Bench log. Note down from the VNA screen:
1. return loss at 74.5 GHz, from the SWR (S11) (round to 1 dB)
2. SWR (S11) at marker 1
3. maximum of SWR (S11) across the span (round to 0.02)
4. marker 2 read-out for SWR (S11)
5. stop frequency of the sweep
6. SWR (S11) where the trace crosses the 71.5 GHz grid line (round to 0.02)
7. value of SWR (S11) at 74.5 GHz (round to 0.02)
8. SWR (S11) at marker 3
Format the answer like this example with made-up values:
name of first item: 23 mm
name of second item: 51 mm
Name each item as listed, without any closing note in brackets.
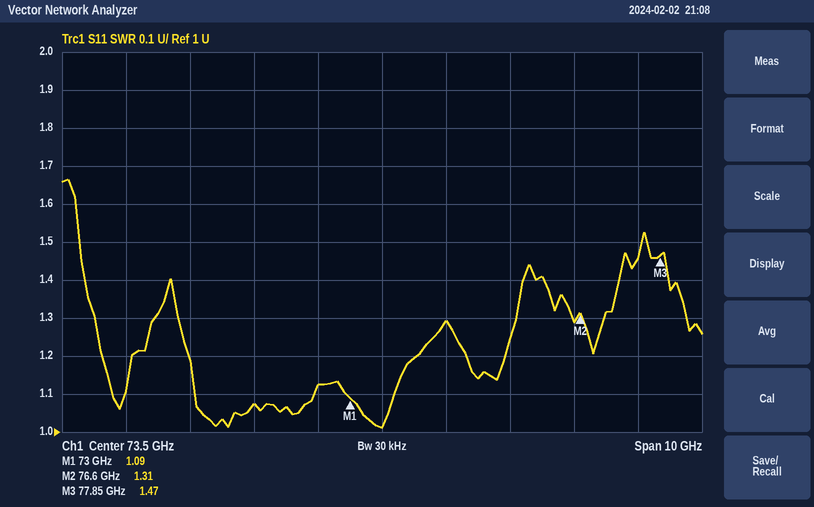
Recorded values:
return loss at 74.5 GHz, from the SWR (S11): 18 dB
SWR (S11) at marker 1: 1.09
maximum of SWR (S11) across the span: 1.66
marker 2 read-out for SWR: 1.31
stop frequency of the sweep: 78.5 GHz
SWR (S11) where the trace crosses the 71.5 GHz grid line: 1.08
value of SWR (S11) at 74.5 GHz: 1.30
SWR (S11) at marker 3: 1.47
